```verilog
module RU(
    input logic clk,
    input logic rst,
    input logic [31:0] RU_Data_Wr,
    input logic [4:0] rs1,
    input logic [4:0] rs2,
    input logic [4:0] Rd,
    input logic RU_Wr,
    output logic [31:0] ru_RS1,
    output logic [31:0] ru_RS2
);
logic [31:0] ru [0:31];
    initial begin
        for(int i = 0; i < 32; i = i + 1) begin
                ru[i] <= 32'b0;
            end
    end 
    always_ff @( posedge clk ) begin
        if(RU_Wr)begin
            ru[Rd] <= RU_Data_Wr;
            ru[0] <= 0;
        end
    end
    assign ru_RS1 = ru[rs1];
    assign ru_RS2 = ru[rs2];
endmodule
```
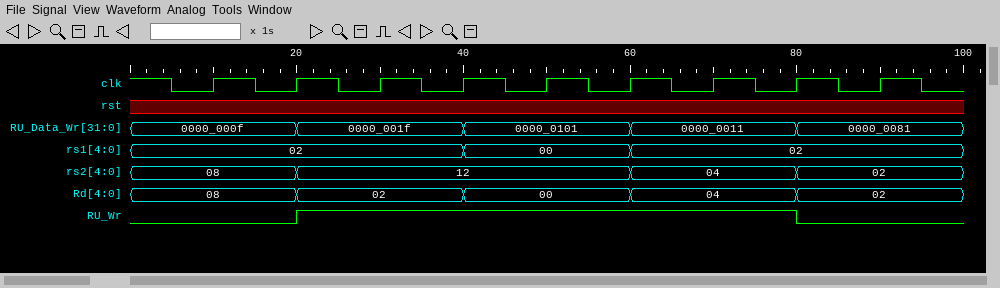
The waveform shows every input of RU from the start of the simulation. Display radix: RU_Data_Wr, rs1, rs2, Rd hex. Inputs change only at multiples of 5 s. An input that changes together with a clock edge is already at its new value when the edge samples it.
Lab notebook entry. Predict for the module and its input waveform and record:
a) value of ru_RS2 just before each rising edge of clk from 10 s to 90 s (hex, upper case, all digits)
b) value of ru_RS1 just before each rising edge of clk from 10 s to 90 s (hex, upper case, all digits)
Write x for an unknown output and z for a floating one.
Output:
00000000, 00000000, 00000000, 00000000, 00000000, 00000000, 00000011, 00000011, 0000001F
00000000, 00000000, 0000001F, 0000001F, 00000000, 00000000, 0000001F, 0000001F, 0000001F
